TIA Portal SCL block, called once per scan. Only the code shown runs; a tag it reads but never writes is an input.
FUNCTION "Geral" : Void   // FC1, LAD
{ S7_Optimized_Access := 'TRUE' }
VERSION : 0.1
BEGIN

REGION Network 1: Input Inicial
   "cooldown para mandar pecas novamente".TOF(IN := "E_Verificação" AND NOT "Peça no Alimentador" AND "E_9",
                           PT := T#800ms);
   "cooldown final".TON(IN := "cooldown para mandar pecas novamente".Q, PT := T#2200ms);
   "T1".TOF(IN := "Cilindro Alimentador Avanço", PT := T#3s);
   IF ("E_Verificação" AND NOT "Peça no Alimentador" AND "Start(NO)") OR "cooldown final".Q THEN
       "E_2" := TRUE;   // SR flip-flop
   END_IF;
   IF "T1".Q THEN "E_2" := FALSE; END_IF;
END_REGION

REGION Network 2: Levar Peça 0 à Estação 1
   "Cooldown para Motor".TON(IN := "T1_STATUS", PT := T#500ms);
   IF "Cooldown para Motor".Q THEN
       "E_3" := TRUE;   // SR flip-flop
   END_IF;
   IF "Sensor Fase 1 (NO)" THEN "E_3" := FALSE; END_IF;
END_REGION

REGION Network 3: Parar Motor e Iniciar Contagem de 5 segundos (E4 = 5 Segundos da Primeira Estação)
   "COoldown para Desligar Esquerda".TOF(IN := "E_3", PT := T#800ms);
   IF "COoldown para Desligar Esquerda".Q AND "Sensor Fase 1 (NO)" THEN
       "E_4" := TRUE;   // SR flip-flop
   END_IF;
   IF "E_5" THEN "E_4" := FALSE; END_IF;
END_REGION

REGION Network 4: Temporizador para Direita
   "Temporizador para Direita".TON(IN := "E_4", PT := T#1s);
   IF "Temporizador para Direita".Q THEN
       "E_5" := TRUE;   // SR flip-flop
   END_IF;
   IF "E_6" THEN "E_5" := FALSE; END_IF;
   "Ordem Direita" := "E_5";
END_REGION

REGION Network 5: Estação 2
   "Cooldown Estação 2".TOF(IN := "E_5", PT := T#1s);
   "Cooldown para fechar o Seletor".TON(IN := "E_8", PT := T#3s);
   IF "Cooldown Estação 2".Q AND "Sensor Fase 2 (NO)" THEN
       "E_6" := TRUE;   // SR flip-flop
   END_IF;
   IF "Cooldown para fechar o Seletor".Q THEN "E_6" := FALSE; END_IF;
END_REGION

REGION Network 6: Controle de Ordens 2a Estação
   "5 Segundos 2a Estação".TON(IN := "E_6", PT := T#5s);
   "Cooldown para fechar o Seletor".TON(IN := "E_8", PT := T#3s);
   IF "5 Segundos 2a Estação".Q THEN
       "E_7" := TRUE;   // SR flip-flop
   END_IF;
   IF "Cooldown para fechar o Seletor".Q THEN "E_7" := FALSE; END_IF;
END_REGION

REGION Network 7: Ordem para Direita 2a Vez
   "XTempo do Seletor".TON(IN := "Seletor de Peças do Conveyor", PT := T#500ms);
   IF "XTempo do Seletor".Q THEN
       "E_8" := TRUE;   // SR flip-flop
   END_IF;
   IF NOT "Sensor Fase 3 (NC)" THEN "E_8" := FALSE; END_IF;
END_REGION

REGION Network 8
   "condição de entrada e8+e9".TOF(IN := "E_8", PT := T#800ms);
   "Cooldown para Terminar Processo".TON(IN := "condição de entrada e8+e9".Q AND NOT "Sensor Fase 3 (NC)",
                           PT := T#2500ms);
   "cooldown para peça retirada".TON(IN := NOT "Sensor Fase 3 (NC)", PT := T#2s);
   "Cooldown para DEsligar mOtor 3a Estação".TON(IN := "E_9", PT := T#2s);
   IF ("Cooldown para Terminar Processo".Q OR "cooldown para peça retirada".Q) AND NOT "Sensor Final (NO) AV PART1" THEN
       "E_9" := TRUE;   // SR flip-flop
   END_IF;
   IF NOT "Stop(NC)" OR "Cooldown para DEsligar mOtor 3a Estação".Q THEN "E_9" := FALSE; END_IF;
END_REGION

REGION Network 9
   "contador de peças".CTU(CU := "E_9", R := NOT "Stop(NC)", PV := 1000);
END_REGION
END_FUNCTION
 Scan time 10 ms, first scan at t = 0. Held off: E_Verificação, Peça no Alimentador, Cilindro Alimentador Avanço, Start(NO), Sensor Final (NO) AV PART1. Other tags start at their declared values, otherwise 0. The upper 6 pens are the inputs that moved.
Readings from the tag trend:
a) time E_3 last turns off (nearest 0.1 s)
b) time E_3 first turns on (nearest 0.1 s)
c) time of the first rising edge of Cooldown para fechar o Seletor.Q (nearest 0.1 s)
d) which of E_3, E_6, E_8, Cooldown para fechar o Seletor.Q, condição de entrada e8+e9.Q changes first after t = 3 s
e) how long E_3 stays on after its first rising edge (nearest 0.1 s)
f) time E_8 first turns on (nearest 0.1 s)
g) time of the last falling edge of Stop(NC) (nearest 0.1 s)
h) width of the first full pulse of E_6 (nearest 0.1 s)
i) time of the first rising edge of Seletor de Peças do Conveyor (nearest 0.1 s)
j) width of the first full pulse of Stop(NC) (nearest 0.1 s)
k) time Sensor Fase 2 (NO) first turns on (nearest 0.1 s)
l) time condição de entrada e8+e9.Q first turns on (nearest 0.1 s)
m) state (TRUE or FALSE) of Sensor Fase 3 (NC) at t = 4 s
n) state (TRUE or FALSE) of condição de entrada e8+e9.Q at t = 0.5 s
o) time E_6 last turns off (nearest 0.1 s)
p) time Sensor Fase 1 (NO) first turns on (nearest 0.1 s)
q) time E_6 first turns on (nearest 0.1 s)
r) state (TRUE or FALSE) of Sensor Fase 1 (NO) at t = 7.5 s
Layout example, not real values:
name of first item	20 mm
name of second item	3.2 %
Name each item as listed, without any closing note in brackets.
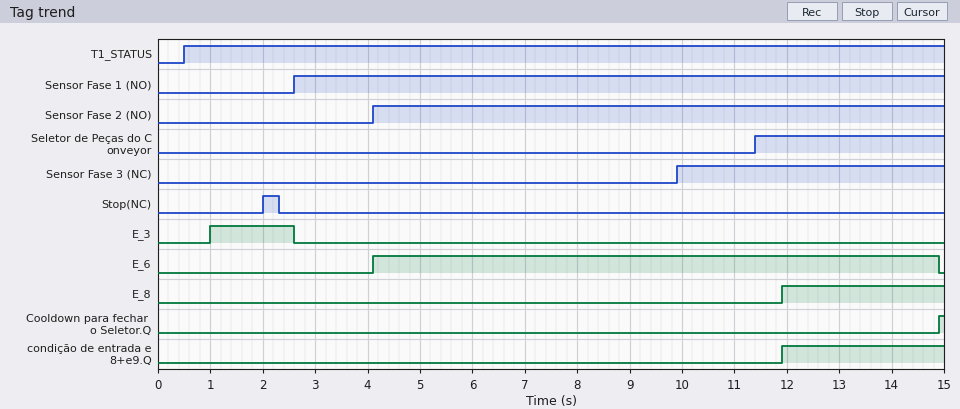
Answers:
time E_3 last turns off	2.6 s
time E_3 first turns on	1.0 s
time of the first rising edge of Cooldown para fechar o Seletor.Q	14.9 s
which of E_3, E_6, E_8, Cooldown para fechar o Seletor.Q, condição de entrada e8+e9.Q changes first after t = 3 s	E_6
how long E_3 stays on after its first rising edge	1.6 s
time E_8 first turns on	11.9 s
time of the last falling edge of Stop(NC)	2.3 s
width of the first full pulse of E_6	10.8 s
time of the first rising edge of Seletor de Peças do Conveyor	11.4 s
width of the first full pulse of Stop(NC)	0.3 s
time Sensor Fase 2 (NO) first turns on	4.1 s
time condição de entrada e8+e9.Q first turns on	11.9 s
state (TRUE or FALSE) of Sensor Fase 3 (NC) at t = 4 s	FALSE
state (TRUE or FALSE) of condição de entrada e8+e9.Q at t = 0.5 s	FALSE
time E_6 last turns off	14.9 s
time Sensor Fase 1 (NO) first turns on	2.6 s
time E_6 first turns on	4.1 s
state (TRUE or FALSE) of Sensor Fase 1 (NO) at t = 7.5 s	TRUE
